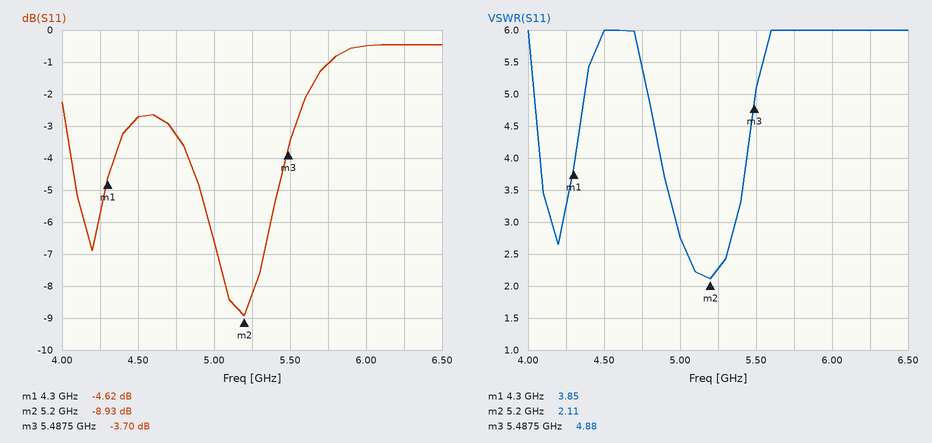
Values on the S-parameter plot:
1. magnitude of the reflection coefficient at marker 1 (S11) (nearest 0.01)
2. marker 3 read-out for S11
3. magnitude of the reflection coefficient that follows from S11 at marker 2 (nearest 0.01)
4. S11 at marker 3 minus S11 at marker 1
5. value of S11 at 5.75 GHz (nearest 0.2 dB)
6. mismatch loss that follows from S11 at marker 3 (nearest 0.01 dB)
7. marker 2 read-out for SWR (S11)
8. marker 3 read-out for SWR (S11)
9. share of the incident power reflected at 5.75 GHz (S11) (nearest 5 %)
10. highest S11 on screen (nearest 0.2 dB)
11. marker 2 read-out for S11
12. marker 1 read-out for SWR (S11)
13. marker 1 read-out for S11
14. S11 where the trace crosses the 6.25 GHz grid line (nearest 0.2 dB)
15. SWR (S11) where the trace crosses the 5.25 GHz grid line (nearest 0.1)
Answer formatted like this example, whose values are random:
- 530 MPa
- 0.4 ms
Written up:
- 0.59
- -3.70 dB
- 0.36
- 0.92 dB
- -1.0 dB
- 2.42 dB
- 2.11
- 4.88
- 80 %
- -0.4 dB
- -8.93 dB
- 3.85
- -4.62 dB
- -0.4 dB
- 2.3
